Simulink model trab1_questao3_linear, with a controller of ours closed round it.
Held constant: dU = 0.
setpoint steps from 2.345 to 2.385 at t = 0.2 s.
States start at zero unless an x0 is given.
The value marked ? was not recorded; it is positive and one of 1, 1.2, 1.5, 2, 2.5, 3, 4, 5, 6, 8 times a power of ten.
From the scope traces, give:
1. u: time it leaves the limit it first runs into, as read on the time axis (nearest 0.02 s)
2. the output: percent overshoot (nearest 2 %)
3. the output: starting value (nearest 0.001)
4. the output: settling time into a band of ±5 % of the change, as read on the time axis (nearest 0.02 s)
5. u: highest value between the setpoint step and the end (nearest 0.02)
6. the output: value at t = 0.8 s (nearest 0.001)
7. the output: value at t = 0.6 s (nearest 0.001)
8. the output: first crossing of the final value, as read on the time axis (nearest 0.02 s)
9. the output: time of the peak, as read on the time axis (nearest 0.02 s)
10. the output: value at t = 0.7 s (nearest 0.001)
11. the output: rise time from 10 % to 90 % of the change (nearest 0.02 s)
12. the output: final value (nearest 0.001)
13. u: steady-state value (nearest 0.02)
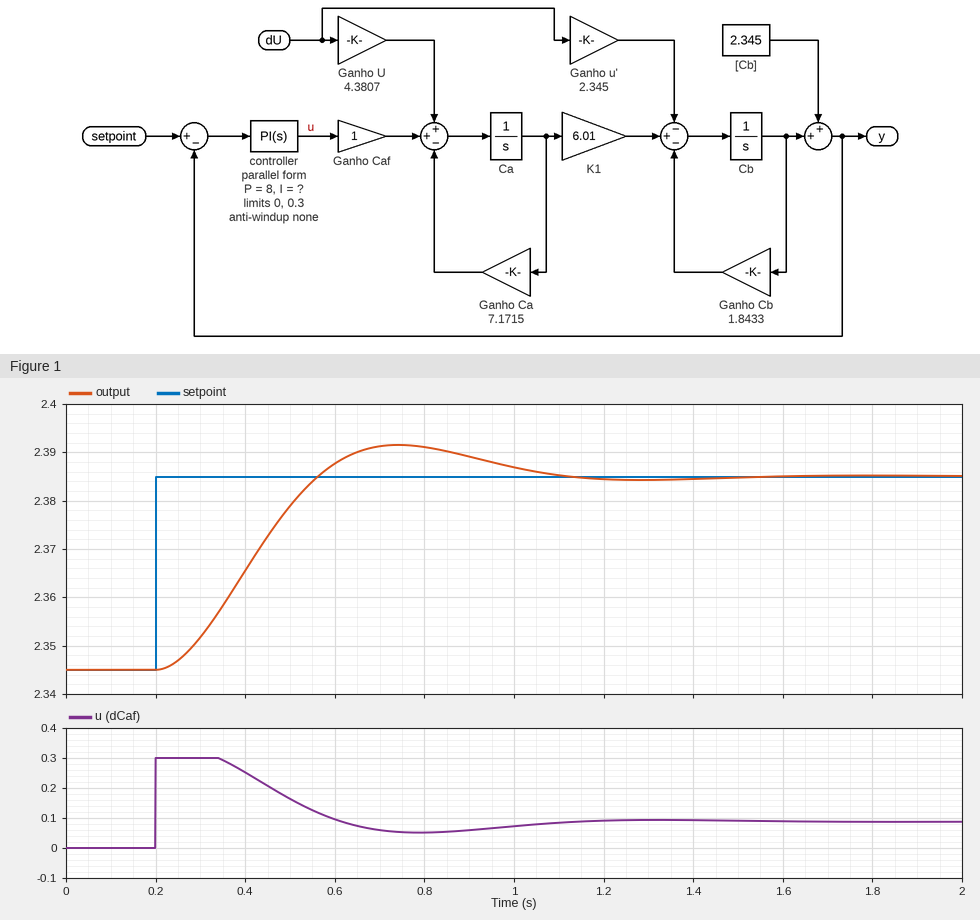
0.34 s
16 %
2.345
1.00 s
0.30
2.391
2.388
0.56 s
0.74 s
2.391
0.24 s
2.385
0.08
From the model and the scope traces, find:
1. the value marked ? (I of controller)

15
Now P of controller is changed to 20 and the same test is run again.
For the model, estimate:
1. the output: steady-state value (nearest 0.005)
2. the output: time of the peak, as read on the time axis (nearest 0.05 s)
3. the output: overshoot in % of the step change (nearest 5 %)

2.385
0.65 s
20 %
